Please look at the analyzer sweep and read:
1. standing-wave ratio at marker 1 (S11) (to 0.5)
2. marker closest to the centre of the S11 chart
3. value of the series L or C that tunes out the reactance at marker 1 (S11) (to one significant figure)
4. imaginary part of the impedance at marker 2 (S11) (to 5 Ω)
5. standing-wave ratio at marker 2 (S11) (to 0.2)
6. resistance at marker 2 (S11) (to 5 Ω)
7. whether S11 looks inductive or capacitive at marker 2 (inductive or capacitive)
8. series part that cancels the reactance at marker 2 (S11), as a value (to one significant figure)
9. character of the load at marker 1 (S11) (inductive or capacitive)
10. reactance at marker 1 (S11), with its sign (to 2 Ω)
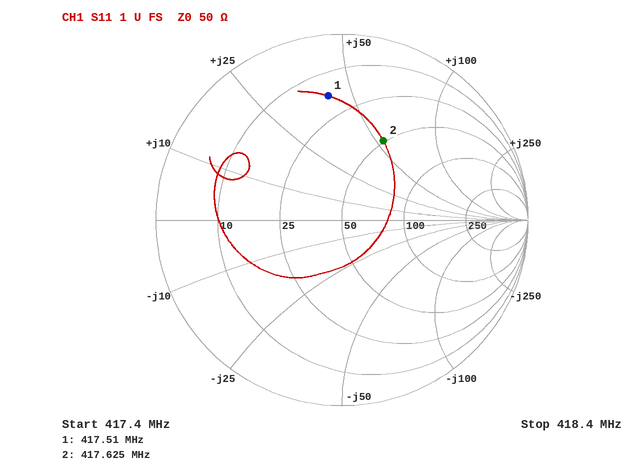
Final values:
5.0
marker 2
9 pF
+55 Ω
2.8
50 Ω
inductive
7 pF
inductive
+42 Ω
